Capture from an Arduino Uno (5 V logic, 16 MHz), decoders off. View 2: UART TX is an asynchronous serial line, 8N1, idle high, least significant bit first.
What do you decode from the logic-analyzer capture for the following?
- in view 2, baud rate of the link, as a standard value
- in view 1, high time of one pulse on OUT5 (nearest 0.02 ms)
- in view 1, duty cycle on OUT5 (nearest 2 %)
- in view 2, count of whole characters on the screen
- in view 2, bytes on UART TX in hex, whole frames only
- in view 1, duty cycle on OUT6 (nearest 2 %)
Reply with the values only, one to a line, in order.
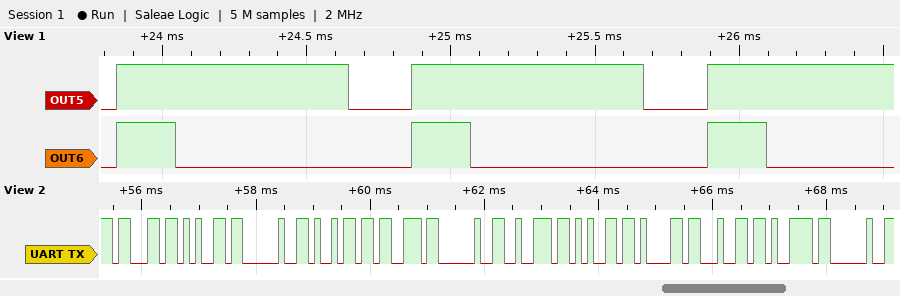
9600 baud
0.80 ms
78 %
12
63 65 20 69 73 20 72 65 61 64 79 20
20 %
